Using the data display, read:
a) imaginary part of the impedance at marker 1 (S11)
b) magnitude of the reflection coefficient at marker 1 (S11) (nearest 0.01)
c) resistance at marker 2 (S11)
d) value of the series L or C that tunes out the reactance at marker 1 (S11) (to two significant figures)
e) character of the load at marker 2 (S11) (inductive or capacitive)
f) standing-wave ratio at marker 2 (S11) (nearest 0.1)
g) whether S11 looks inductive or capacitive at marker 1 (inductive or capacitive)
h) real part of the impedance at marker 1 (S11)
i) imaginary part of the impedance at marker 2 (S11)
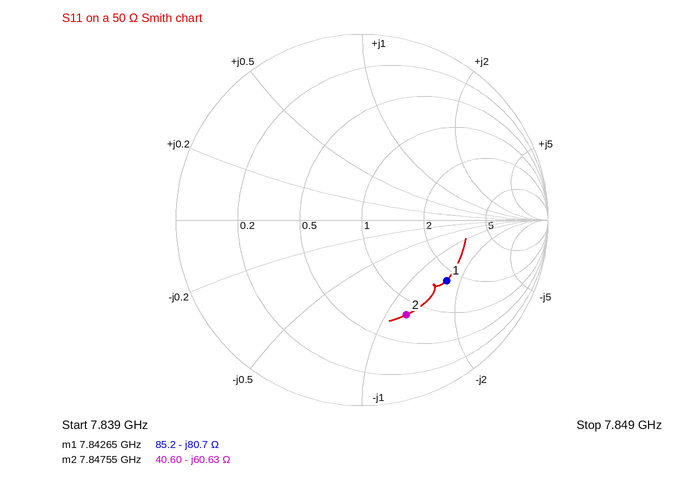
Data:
-80.7 Ω
0.56
40.60 Ω
1.6 nH
capacitive
3.6
capacitive
85.2 Ω
-60.63 Ω
